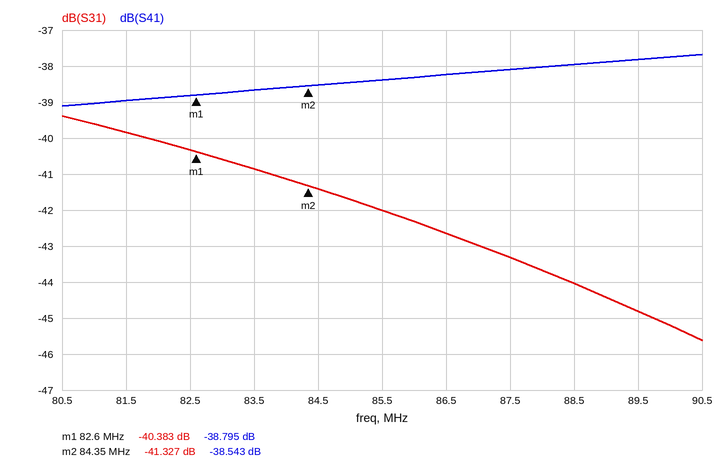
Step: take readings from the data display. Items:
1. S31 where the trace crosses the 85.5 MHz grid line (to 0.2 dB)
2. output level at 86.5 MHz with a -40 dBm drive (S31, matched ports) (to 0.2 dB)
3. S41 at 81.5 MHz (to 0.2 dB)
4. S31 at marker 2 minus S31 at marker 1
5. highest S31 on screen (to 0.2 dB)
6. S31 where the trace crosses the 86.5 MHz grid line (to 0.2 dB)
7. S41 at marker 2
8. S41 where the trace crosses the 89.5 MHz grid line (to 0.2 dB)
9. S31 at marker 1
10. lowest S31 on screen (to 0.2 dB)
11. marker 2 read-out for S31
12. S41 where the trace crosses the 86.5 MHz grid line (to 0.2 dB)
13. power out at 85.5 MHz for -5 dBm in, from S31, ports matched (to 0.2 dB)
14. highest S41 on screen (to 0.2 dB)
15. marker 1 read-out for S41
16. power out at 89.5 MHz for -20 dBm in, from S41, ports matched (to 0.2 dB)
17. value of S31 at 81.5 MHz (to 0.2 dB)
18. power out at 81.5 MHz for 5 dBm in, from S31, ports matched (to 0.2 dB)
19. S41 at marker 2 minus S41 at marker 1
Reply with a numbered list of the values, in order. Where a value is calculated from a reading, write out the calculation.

1. -42.0 dB
2. -40 dBm + (-42.6 dB) = -82.6 dBm
3. -39.0 dB
4. -41.327 − (-40.383) = -0.944 dB
5. -39.4 dB
6. -42.6 dB
7. -38.543 dB
8. -37.8 dB
9. -40.383 dB
10. -45.6 dB
11. -41.327 dB
12. -38.2 dB
13. -5 dBm + (-42.0 dB) = -47.0 dBm
14. -37.6 dB
15. -38.795 dB
16. -20 dBm + (-37.8 dB) = -57.8 dBm
17. -39.8 dB
18. 5 dBm + (-39.8 dB) = -34.8 dBm
19. -38.543 − (-38.795) = 0.252 dB
